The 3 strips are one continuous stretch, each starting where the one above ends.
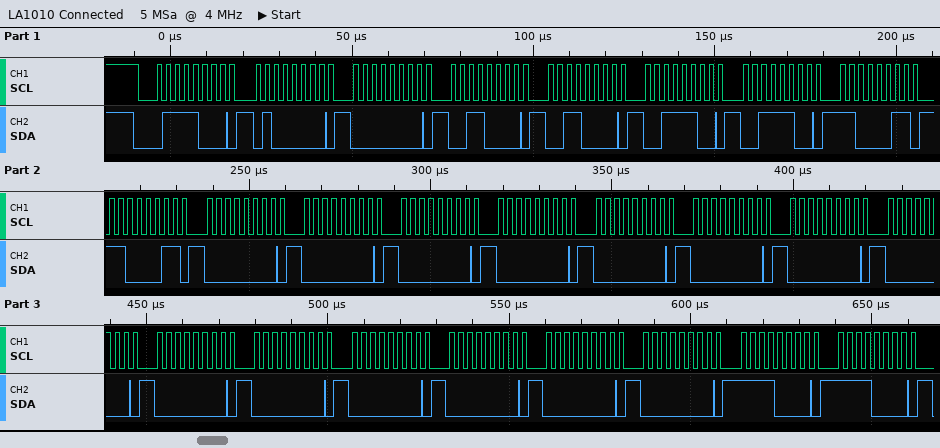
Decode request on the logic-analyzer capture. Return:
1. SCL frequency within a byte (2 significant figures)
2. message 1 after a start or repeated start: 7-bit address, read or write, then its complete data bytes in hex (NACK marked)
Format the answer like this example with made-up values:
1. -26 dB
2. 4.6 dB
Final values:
1. 400 kHz
2. 0x3C write: 40 00 30 30 3C 3C C3 C3 00 00 00 00 00 00 00 00 00 00 00 00 00 00 F0 F0
